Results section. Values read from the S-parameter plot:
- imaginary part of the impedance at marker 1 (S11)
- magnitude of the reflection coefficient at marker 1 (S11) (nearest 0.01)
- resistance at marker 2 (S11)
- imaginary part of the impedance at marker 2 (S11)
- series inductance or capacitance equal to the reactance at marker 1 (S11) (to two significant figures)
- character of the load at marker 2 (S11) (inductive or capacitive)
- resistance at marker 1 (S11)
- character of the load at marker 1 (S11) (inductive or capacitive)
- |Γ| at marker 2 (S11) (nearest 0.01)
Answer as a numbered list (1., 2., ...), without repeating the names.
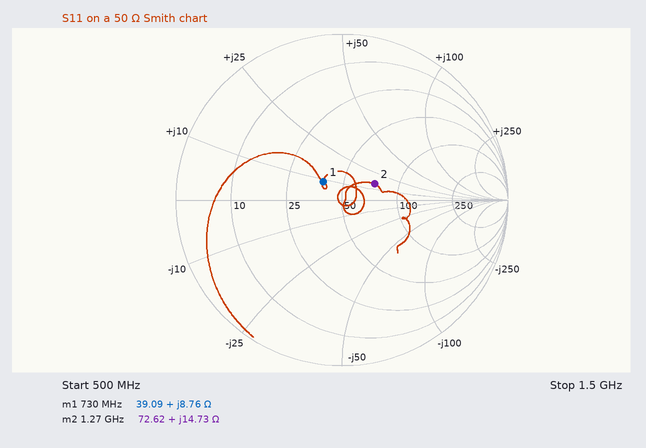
1. +8.76 Ω
2. 0.16
3. 72.62 Ω
4. +14.73 Ω
5. 1.9 nH
6. inductive
7. 39.09 Ω
8. inductive
9. 0.22
